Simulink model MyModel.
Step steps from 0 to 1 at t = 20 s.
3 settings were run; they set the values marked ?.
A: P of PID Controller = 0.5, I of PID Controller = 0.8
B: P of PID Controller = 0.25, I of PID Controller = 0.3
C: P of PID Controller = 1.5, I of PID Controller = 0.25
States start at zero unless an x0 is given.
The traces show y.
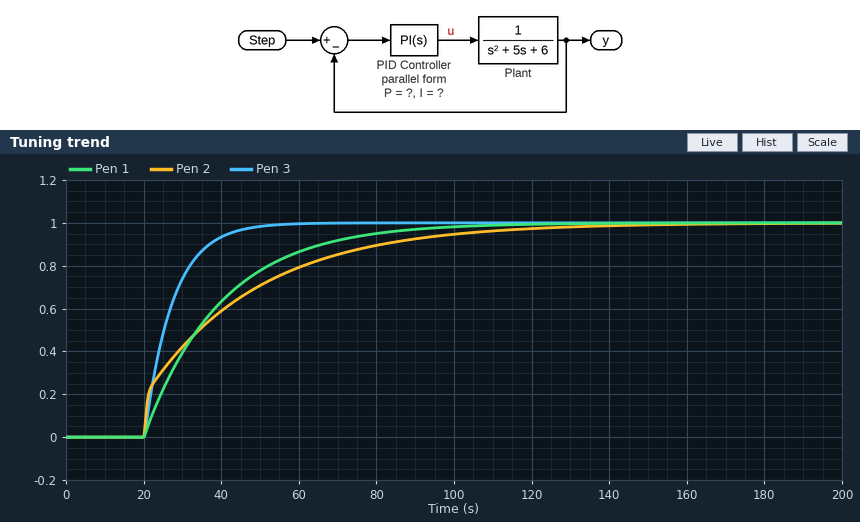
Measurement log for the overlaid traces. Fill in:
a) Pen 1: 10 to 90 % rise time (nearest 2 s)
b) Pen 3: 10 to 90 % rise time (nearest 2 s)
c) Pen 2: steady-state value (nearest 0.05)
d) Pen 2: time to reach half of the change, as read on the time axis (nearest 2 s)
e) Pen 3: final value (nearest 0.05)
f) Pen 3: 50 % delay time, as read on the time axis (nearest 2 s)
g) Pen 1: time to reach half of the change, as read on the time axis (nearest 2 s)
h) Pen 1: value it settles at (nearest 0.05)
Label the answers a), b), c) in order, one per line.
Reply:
a) 44 s
b) 16 s
c) 1.00
d) 34 s
e) 1.00
f) 26 s
g) 34 s
h) 1.00
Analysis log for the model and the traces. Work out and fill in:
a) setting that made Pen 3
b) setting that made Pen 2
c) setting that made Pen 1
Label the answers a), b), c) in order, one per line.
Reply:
a) A
b) C
c) B
